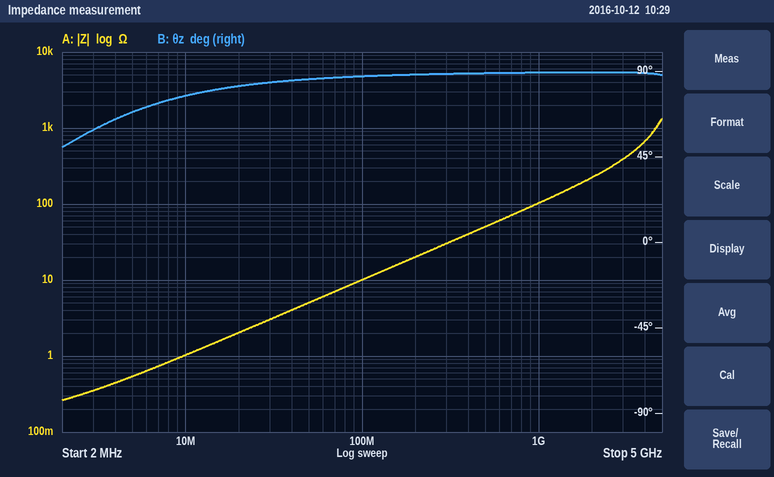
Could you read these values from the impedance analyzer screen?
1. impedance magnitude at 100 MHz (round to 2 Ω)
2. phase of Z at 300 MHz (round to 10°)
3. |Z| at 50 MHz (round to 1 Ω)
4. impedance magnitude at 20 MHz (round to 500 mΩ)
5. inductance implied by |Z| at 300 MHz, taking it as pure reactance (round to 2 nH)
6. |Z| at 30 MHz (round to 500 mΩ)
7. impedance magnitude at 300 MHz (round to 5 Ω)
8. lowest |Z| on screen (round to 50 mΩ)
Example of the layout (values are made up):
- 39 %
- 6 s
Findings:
- 10 Ω
- 90°
- 5 Ω
- 2.0 Ω
- 16 nH
- 3.0 Ω
- 30 Ω
- 250 mΩ
